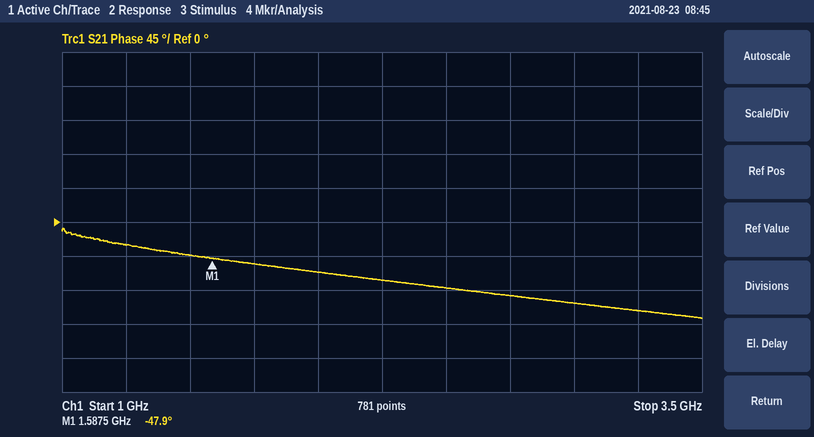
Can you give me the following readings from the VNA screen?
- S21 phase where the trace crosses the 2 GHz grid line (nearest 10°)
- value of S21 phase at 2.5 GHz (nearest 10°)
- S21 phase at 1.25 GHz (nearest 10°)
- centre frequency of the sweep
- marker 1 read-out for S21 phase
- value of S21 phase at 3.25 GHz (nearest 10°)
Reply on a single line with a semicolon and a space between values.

-70°; -90°; -30°; 2.25 GHz; -47.9°; -120°
